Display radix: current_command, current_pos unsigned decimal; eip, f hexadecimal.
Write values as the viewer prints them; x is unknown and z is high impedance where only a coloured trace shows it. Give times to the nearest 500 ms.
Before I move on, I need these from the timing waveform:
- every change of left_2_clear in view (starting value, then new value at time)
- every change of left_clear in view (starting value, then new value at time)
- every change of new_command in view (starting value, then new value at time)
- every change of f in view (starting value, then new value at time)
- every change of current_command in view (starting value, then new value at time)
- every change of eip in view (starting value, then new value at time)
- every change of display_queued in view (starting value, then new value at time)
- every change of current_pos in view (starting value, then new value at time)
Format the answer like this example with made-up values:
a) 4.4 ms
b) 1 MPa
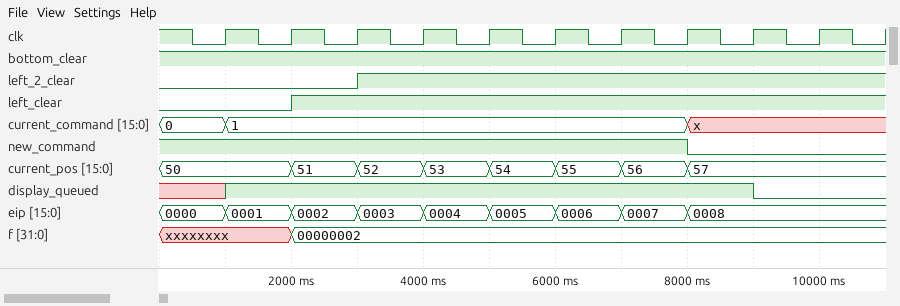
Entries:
a) 0, 1 at 3000 ms
b) 0, 1 at 2000 ms
c) 1, 0 at 8000 ms
d) xxxxxxxx, 00000002 at 2000 ms
e) 0, 1 at 1000 ms, x at 8000 ms
f) 0000, 0001 at 1000 ms, 0002 at 2000 ms, 0003 at 3000 ms, 0004 at 4000 ms, 0005 at 5000 ms, 0006 at 6000 ms, 0007 at 7000 ms, 0008 at 8000 ms
g) x, 1 at 1000 ms, 0 at 9000 ms
h) 50, 51 at 2000 ms, 52 at 3000 ms, 53 at 4000 ms, 54 at 5000 ms, 55 at 6000 ms, 56 at 7000 ms, 57 at 8000 ms
